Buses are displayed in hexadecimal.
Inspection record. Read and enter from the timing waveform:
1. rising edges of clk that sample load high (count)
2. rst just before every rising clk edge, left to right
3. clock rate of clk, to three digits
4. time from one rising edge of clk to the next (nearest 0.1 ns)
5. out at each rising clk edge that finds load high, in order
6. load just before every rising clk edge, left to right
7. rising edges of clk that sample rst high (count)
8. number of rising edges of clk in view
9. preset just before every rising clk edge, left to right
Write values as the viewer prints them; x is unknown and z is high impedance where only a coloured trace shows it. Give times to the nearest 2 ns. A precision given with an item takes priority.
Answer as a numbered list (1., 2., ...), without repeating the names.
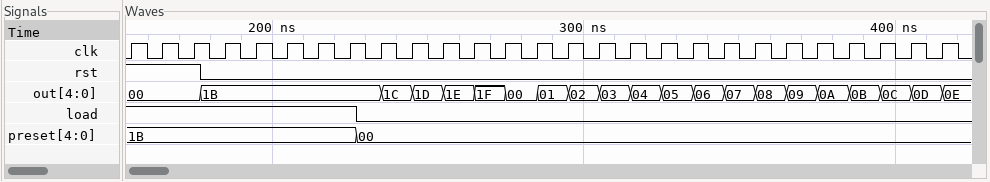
1. 8
2. 1 1 1 0 0 0 0 0 0 0 0 0 0 0 0 0 0 0 0 0 0 0 0 0 0 0 0
3. 100 MHz
4. 10 ns
5. 00, 00, 00, 1B, 1B, 1B, 1B, 1B
6. 1 1 1 1 1 1 1 1 0 0 0 0 0 0 0 0 0 0 0 0 0 0 0 0 0 0 0
7. 3
8. 27
9. 1B, 1B, 1B, 1B, 1B, 1B, 1B, 1B, 00, 00, 00, 00, 00, 00, 00, 00, 00, 00, 00, 00, 00, 00, 00, 00, 00, 00, 00
